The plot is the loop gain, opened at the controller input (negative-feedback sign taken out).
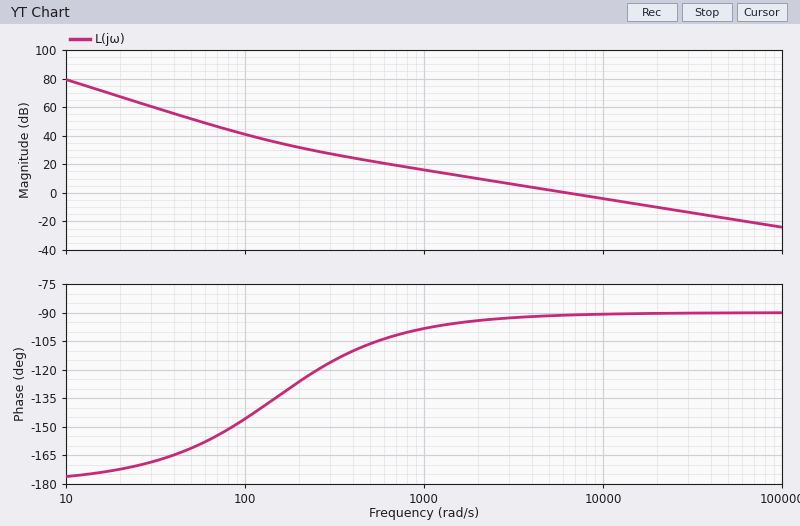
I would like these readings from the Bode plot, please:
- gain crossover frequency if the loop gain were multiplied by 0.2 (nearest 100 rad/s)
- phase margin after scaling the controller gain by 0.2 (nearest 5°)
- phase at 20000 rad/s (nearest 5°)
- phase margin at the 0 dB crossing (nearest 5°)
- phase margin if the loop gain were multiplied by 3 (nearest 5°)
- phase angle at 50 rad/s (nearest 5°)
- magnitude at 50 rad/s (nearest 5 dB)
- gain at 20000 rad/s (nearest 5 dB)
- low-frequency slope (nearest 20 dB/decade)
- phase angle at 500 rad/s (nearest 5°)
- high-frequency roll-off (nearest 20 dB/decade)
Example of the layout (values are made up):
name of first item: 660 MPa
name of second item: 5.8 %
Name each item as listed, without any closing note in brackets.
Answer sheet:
gain crossover frequency if the loop gain were multiplied by 0.2: 1300 rad/s
phase margin after scaling the controller gain by 0.2: 85°
phase at 20000 rad/s: -90°
phase margin at the 0 dB crossing: 90°
phase margin if the loop gain were multiplied by 3: 90°
phase angle at 50 rad/s: -160°
magnitude at 50 rad/s: 50 dB
gain at 20000 rad/s: -10 dB
low-frequency slope: -40 dB/decade
phase angle at 500 rad/s: -105°
high-frequency roll-off: -20 dB/decade
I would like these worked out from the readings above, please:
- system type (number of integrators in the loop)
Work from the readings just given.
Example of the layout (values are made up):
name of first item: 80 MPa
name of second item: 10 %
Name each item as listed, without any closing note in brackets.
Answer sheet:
system type: 2
